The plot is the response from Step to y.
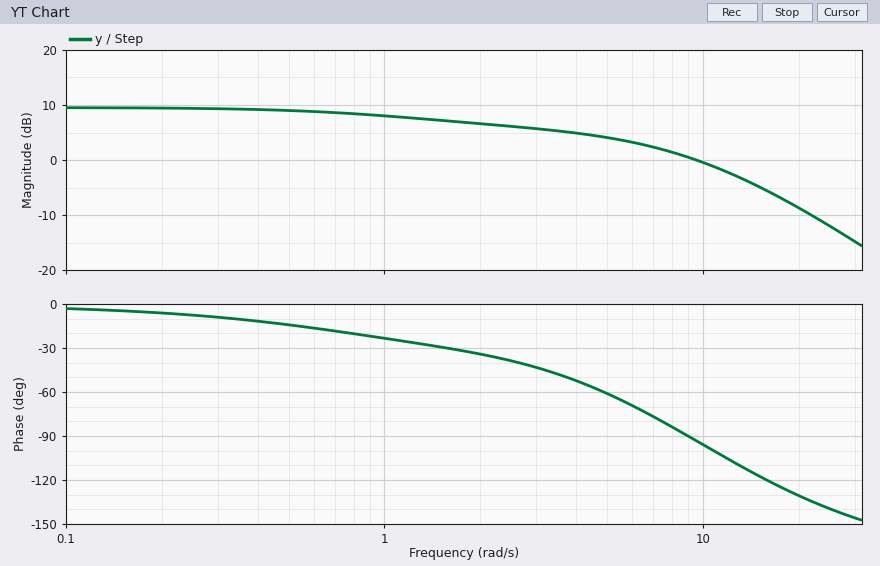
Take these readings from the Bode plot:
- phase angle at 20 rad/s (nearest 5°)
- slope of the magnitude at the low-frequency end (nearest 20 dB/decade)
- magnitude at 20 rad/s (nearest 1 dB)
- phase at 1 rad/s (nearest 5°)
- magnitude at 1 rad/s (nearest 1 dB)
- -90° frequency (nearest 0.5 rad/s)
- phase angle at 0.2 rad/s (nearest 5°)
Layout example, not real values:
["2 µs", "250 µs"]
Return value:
["-130°", "0 dB/decade", "-9 dB", "-25°", "8 dB", "9.0 rad/s", "-5°"]
